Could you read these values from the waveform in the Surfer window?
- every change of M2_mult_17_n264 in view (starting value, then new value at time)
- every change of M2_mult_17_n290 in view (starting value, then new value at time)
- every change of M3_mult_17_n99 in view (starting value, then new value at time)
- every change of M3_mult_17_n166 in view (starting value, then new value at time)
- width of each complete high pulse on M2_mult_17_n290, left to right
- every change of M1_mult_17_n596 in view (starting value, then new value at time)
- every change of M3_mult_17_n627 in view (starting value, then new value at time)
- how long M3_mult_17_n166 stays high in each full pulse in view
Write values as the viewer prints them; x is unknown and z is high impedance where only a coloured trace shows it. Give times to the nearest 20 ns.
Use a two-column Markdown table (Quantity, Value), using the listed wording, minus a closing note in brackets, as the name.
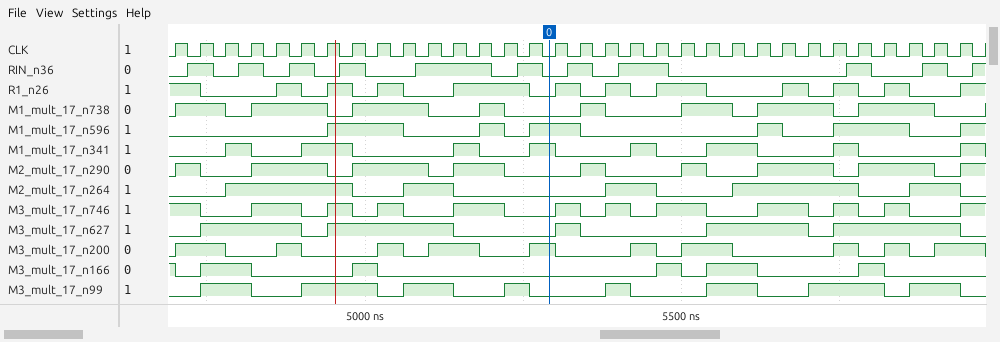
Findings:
| Quantity | Value |
|---|---|
| every change of M2_mult_17_n264 in view | 0, 1 at 4780 ns, 0 at 4980 ns, 1 at 5060 ns, 0 at 5140 ns, 1 at 5380 ns, 0 at 5460 ns, 1 at 5580 ns, 0 at 5780 ns, 1 at 5860 ns, 0 at 5940 ns |
| every change of M2_mult_17_n290 in view | 0, 1 at 4700 ns, 0 at 4740 ns, 1 at 4820 ns, 0 at 4940 ns, 1 at 4980 ns, 0 at 5100 ns, 1 at 5140 ns, 0 at 5220 ns, 1 at 5340 ns, 0 at 5380 ns, 1 at 5500 ns, 0 at 5540 ns, 1 at 5620 ns, 0 at 5740 ns, 1 at 5780 ns, 0 at 5900 ns, 1 at 5940 ns |
| every change of M3_mult_17_n99 in view | 0, 1 at 4740 ns, 0 at 4820 ns, 1 at 4900 ns, 0 at 5020 ns, 1 at 5060 ns, 0 at 5140 ns, 1 at 5220 ns, 0 at 5260 ns, 1 at 5380 ns, 0 at 5420 ns, 1 at 5540 ns, 0 at 5620 ns, 1 at 5700 ns, 0 at 5820 ns, 1 at 5860 ns, 0 at 5940 ns |
| every change of M3_mult_17_n166 in view | 1, 0 at 4700 ns, 1 at 4740 ns, 0 at 4820 ns, 1 at 4980 ns, 0 at 5020 ns, 1 at 5460 ns, 0 at 5500 ns, 1 at 5540 ns, 0 at 5620 ns, 1 at 5780 ns, 0 at 5820 ns |
| width of each complete high pulse on M2_mult_17_n290, left to right | 40 ns, 120 ns, 120 ns, 80 ns, 40 ns, 40 ns, 120 ns, 120 ns |
| every change of M1_mult_17_n596 in view | 0, 1 at 4940 ns, 0 at 5060 ns, 1 at 5180 ns, 0 at 5220 ns, 1 at 5260 ns, 0 at 5340 ns, 1 at 5620 ns, 0 at 5660 ns, 1 at 5740 ns, 0 at 5860 ns, 1 at 5940 ns |
| every change of M3_mult_17_n627 in view | 0, 1 at 4740 ns, 0 at 4900 ns, 1 at 4940 ns, 0 at 5140 ns, 1 at 5300 ns, 0 at 5340 ns, 1 at 5540 ns, 0 at 5700 ns, 1 at 5740 ns, 0 at 5940 ns |
| how long M3_mult_17_n166 stays high in each full pulse in view | 80 ns, 40 ns, 40 ns, 80 ns, 40 ns |
